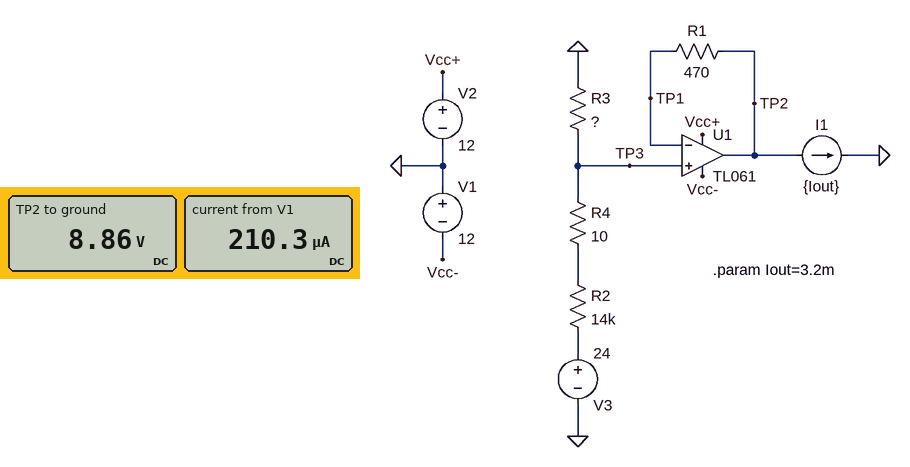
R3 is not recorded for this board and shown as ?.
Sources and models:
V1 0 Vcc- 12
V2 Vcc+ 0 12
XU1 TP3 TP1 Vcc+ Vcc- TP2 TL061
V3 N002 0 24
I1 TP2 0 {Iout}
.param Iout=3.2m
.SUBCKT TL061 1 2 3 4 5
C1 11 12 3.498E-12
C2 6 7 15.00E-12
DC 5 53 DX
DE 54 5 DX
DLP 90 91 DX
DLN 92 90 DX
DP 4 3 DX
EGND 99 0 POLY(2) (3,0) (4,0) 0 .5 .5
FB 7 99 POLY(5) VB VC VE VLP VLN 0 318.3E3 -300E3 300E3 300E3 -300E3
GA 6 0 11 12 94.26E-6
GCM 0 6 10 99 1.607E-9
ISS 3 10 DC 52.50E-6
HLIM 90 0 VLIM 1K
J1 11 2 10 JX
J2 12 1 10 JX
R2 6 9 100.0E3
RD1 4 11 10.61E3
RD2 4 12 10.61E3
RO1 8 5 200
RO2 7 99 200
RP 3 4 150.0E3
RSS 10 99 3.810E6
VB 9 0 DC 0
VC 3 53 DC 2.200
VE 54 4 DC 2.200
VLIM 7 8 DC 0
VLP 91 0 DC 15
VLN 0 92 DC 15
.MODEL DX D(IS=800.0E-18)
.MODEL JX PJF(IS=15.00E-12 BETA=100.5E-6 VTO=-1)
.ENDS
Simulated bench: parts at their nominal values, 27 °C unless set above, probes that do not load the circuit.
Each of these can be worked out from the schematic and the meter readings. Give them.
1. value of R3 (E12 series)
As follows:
8.2 kΩ
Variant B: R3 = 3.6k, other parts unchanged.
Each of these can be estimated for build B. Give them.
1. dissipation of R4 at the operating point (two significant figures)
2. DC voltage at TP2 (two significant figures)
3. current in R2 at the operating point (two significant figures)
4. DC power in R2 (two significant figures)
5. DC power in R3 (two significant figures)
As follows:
19 µW
4.9 V
1.4 mA
26 mW
6.7 mW
